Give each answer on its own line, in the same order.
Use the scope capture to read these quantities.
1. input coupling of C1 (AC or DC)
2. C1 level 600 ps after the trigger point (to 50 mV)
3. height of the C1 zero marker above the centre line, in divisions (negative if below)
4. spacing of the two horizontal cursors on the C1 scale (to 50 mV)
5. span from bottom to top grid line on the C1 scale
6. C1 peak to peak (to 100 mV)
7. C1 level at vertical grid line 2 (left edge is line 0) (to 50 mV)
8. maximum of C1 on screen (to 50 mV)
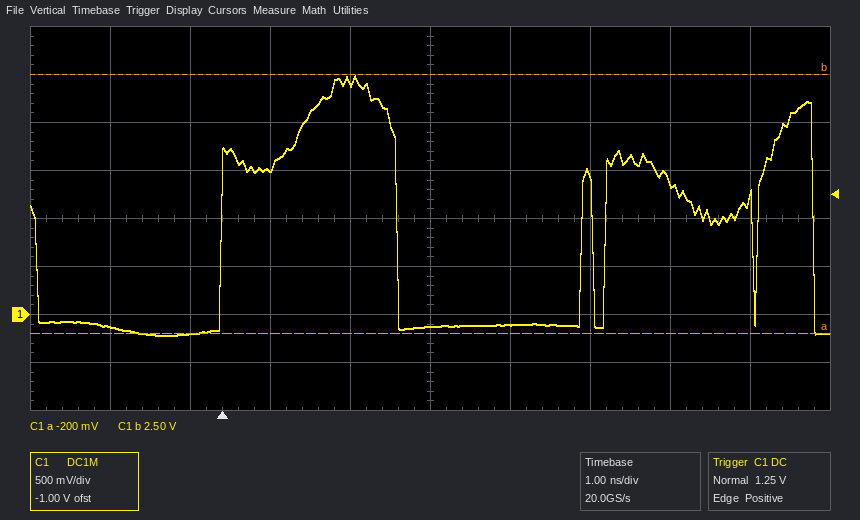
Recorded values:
DC
1.55 V
-2.0 div
2.70 V
4 V
2.70 V
-200 mV
2.50 V
